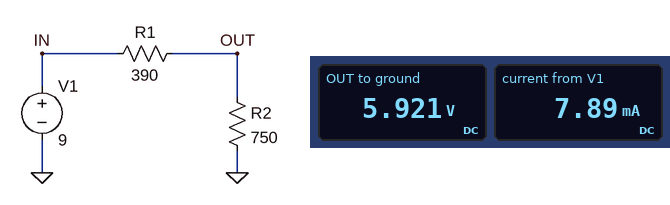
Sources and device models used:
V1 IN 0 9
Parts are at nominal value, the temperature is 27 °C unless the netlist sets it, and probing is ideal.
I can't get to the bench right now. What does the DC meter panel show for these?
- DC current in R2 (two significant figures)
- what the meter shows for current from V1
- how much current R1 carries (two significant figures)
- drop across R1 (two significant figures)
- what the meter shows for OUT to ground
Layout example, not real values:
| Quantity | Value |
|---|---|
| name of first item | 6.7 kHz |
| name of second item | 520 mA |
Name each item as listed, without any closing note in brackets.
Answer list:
| Quantity | Value |
|---|---|
| DC current in R2 | 7.9 mA |
| what the meter shows for current from V1 | 7.89 mA |
| how much current R1 carries | 7.9 mA |
| drop across R1 | 3.1 V |
| what the meter shows for OUT to ground | 5.921 V |
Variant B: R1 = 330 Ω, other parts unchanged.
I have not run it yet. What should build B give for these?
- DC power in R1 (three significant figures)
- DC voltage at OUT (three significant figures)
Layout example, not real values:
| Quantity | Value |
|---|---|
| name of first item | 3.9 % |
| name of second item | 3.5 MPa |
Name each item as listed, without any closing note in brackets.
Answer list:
| Quantity | Value |
|---|---|
| DC power in R1 | 22.9 mW |
| DC voltage at OUT | 6.25 V |
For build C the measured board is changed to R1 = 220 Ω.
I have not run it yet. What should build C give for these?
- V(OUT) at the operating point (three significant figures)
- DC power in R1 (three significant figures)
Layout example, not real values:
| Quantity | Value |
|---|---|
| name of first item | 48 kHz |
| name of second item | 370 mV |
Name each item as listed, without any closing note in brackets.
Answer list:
| Quantity | Value |
|---|---|
| V(OUT) at the operating point | 6.96 V |
| DC power in R1 | 18.9 mW |
